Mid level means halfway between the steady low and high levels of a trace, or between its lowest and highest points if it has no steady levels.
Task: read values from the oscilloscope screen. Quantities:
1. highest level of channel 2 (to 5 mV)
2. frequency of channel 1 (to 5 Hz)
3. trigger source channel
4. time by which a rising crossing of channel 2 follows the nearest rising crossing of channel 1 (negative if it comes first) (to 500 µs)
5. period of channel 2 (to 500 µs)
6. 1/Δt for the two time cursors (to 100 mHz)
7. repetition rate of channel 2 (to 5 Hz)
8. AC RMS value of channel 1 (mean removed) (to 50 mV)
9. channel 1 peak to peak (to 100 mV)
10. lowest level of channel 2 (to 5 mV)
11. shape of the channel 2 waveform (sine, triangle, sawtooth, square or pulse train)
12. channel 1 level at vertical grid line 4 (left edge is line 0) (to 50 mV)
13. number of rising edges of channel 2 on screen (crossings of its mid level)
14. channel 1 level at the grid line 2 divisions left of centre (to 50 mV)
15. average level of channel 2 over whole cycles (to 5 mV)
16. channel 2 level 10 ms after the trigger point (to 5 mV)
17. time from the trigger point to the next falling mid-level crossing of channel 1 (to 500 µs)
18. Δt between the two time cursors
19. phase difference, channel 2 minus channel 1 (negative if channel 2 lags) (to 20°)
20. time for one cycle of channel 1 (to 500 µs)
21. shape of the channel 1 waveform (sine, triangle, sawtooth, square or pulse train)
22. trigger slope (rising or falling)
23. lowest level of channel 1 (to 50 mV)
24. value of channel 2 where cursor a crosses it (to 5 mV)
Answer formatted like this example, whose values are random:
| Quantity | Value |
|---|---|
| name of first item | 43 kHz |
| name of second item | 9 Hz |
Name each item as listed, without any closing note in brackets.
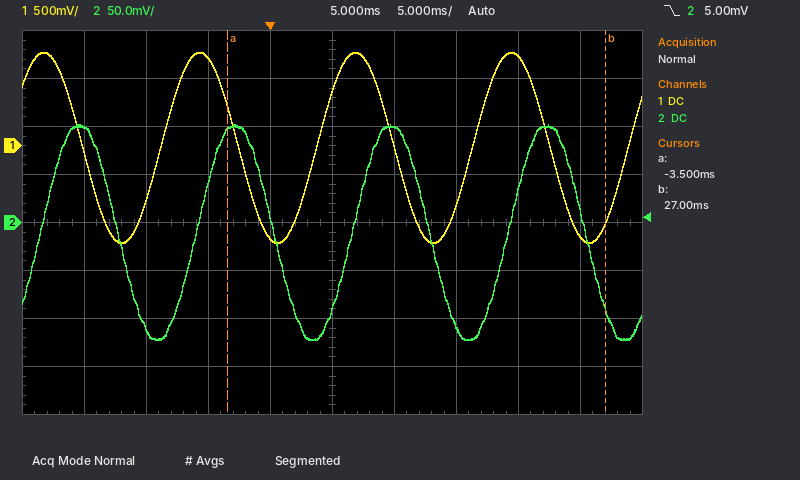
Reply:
| Quantity | Value |
|---|---|
| highest level of channel 2 | 100 mV |
| frequency of channel 1 | 80 Hz |
| trigger source channel | channel 2 |
| time by which a rising crossing of channel 2 follows the nearest rising crossing of channel 1 (negative if it comes first) | +3.0 ms |
| period of channel 2 | 12.5 ms |
| 1/Δt for the two time cursors | 32.8 Hz |
| repetition rate of channel 2 | 80 Hz |
| AC RMS value of channel 1 (mean removed) | 700 mV |
| channel 1 peak to peak | 2.00 V |
| lowest level of channel 2 | -120 mV |
| shape of the channel 2 waveform | sine |
| channel 1 level at vertical grid line 4 (left edge is line 0) | -950 mV |
| number of rising edges of channel 2 on screen | 4 |
| channel 1 level at the grid line 2 divisions left of centre | 900 mV |
| average level of channel 2 over whole cycles | -10 mV |
| channel 2 level 10 ms after the trigger point | 100 mV |
| time from the trigger point to the next falling mid-level crossing of channel 1 | 10.0 ms |
| Δt between the two time cursors | 30.5 ms |
| phase difference, channel 2 minus channel 1 (negative if channel 2 lags) | -80° |
| time for one cycle of channel 1 | 12.5 ms |
| shape of the channel 1 waveform | sine |
| trigger slope | falling |
| lowest level of channel 1 | -1.00 V |
| value of channel 2 where cursor a crosses it | 95 mV |
